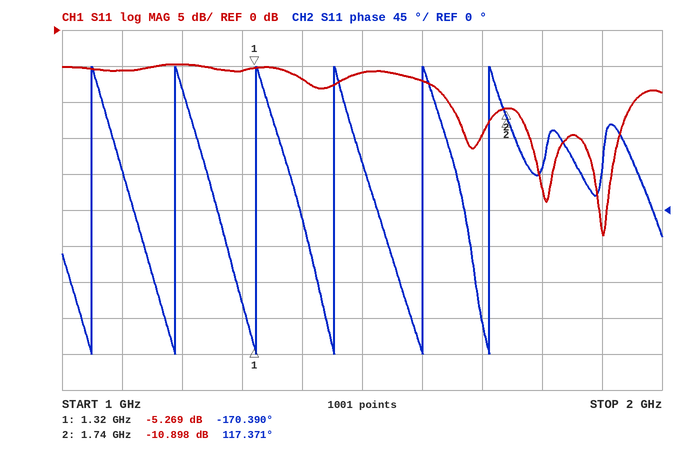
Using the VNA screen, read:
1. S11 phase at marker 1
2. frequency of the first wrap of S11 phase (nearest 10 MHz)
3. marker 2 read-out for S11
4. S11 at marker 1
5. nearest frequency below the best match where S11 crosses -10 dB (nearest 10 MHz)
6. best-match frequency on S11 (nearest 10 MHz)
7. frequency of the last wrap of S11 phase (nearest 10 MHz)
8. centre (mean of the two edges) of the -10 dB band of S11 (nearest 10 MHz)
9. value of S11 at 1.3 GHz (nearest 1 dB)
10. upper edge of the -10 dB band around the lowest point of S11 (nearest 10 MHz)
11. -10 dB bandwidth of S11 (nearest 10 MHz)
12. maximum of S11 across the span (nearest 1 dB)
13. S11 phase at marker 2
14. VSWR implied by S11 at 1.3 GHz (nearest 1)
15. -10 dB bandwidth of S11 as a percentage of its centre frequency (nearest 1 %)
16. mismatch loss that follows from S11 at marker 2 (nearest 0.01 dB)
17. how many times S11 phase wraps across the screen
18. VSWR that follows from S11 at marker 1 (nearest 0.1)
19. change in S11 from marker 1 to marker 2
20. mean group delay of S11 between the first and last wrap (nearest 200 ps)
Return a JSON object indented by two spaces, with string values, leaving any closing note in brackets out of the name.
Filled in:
{
  "S11 phase at marker 1": "-170.390°",
  "frequency of the first wrap of S11 phase": "1.05 GHz",
  "marker 2 read-out for S11": "-10.898 dB",
  "S11 at marker 1": "-5.269 dB",
  "nearest frequency below the best match where S11 crosses -10 dB": "1.64 GHz",
  "best-match frequency on S11": "1.90 GHz",
  "frequency of the last wrap of S11 phase": "1.71 GHz",
  "centre (mean of the two edges) of the -10 dB band of S11": "1.80 GHz",
  "value of S11 at 1.3 GHz": "-6 dB",
  "upper edge of the -10 dB band around the lowest point of S11": "1.95 GHz",
  "-10 dB bandwidth of S11": "310 MHz",
  "maximum of S11 across the span": "-5 dB",
  "S11 phase at marker 2": "117.371°",
  "VSWR implied by S11 at 1.3 GHz": "3",
  "-10 dB bandwidth of S11 as a percentage of its centre frequency": "17 %",
  "mismatch loss that follows from S11 at marker 2": "0.37 dB",
  "how many times S11 phase wraps across the screen": "6",
  "VSWR that follows from S11 at marker 1": "3.4",
  "change in S11 from marker 1 to marker 2": "-5.629 dB",
  "mean group delay of S11 between the first and last wrap": "7.6 ns"
}
